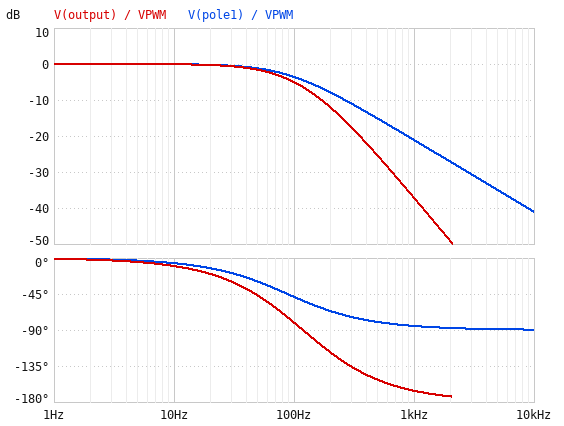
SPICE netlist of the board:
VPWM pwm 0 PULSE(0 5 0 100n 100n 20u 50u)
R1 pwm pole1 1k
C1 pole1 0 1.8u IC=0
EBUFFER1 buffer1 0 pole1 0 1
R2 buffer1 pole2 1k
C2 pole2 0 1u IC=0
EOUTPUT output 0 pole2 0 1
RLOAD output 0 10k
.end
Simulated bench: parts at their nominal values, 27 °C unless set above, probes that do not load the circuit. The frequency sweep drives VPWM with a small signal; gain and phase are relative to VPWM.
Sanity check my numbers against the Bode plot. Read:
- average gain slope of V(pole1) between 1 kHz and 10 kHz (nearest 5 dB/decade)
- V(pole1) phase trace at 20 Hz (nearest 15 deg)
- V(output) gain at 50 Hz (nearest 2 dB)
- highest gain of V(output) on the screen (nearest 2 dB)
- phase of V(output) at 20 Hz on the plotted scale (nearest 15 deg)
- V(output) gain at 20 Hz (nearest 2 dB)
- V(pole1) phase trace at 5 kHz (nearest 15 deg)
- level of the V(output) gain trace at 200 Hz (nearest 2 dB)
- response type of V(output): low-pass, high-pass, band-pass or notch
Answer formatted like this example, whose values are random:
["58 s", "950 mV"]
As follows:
["-20 dB/decade", "-15 deg", "-2 dB", "0 dB", "-15 deg", "0 dB", "-90 deg", "-12 dB", "low-pass"]
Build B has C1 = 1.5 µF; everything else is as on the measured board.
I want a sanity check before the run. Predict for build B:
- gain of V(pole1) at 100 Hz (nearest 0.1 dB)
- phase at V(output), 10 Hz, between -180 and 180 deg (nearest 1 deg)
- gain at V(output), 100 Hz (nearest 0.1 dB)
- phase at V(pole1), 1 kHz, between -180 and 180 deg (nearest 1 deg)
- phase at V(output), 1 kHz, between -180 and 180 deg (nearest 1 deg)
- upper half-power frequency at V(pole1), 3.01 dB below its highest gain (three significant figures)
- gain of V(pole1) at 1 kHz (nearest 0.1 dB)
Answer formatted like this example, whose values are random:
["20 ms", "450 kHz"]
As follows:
["-2.8 dB", "-9 deg", "-4.2 dB", "-84 deg", "-165 deg", "106 Hz", "-19.5 dB"]
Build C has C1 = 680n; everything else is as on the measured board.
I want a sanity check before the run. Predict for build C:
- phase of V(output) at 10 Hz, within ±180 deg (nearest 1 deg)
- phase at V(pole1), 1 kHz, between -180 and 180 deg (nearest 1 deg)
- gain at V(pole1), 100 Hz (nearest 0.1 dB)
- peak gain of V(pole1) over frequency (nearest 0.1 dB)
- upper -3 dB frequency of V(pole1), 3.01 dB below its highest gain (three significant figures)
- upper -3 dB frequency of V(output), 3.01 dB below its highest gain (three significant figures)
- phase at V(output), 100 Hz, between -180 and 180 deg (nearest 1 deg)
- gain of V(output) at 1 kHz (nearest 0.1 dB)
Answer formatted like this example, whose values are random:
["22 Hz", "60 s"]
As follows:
["-6 deg", "-77 deg", "-0.7 dB", "0 dB", "234 Hz", "121 Hz", "-55 deg", "-28.9 dB"]
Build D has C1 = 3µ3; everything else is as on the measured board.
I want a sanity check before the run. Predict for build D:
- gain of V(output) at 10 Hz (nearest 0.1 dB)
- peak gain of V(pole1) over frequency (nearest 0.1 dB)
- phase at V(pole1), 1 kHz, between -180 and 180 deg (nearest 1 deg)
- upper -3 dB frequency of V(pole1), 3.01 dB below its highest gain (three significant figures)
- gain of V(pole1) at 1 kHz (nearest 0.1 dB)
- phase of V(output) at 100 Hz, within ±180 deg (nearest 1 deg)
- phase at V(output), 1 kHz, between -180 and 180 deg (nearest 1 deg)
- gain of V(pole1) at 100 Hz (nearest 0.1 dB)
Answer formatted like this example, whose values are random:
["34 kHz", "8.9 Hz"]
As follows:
["-0.2 dB", "0 dB", "-87 deg", "48.2 Hz", "-26.3 dB", "-96 deg", "-168 deg", "-7.2 dB"]
